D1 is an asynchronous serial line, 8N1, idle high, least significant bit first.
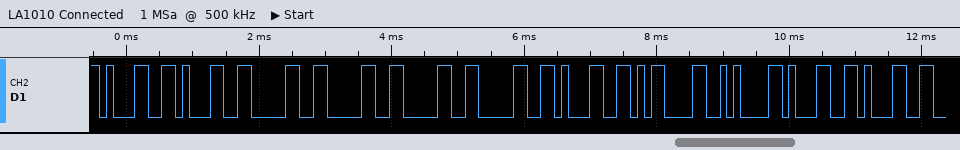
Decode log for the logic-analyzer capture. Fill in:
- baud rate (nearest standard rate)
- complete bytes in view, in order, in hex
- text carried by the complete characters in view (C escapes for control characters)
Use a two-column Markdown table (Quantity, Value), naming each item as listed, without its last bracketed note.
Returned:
| Quantity | Value |
|---|---|
| baud rate | 9600 baud |
| complete bytes in view, in order, in hex | 31 31 30 30 30 30 31 0D 0A 31 31 |
| text carried by the complete characters in view | "1100001\r\n11" |
